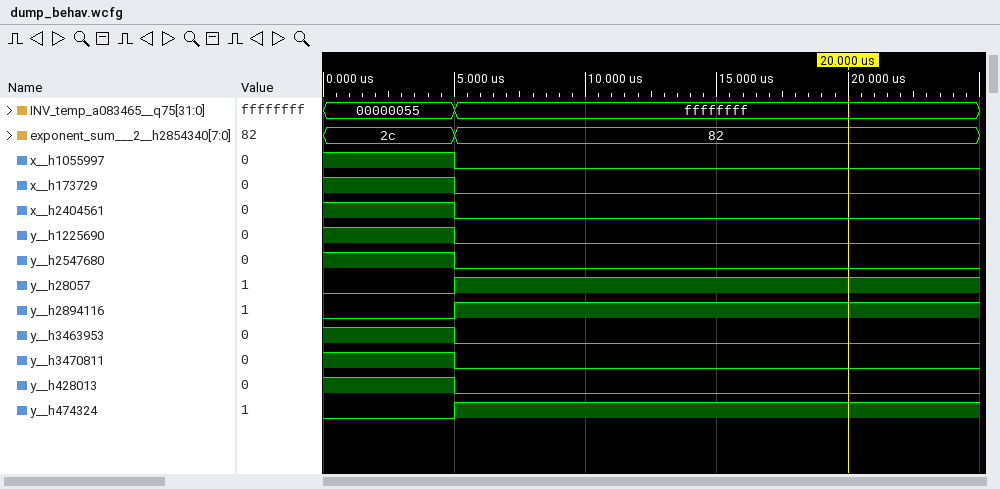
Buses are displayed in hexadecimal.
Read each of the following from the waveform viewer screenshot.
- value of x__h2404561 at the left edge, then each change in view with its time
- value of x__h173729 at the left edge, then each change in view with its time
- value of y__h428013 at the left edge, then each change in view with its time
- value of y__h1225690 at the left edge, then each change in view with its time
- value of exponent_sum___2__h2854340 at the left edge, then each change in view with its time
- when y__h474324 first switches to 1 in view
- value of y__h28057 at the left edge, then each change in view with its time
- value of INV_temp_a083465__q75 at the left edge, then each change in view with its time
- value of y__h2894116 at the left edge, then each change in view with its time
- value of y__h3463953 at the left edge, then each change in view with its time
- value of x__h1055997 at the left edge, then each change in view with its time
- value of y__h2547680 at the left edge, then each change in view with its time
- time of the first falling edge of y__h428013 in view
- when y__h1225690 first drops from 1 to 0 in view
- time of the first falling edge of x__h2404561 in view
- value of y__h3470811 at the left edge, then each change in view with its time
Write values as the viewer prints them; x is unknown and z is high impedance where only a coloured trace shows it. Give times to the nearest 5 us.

1, 0 at 5 us
1, 0 at 5 us
1, 0 at 5 us
1, 0 at 5 us
2c, 82 at 5 us
5 us
0, 1 at 5 us
00000055, ffffffff at 5 us
0, 1 at 5 us
1, 0 at 5 us
1, 0 at 5 us
1, 0 at 5 us
5 us
5 us
5 us
1, 0 at 5 us
